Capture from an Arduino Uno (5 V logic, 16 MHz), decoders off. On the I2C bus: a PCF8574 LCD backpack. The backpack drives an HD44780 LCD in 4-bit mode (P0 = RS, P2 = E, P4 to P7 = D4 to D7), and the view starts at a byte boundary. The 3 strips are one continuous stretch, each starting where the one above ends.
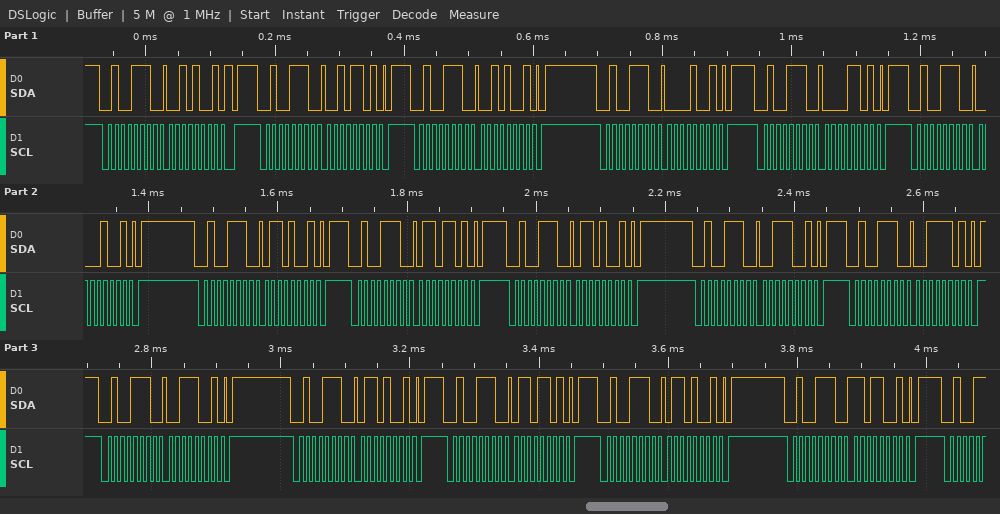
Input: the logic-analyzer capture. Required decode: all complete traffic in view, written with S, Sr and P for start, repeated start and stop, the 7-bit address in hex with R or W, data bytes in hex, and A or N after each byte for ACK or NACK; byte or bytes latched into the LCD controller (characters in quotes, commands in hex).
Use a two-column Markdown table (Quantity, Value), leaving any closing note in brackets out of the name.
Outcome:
| Quantity | Value |
|---|---|
| all complete traffic in view, written with S, Sr and P for start, repeated start and stop, the 7-bit address in hex with R or W, data bytes in hex, and A or N after each byte for ACK or NACK | S 27W A 29 A P S 27W A 2D A P S 27W A 29 A P S 27W A 09 A P S 27W A 0D A P S 27W A 09 A P S 27W A 69 A P S 27W A 6D A P S 27W A 69 A P S 27W A 39 A P S 27W A 3D A P S 27W A 39 A P S 27W A 69 A P S 27W A 6D A P S 27W A 69 A P S 27W A D9 A P |
| byte or bytes latched into the LCD controller | ' ' 'c' |
